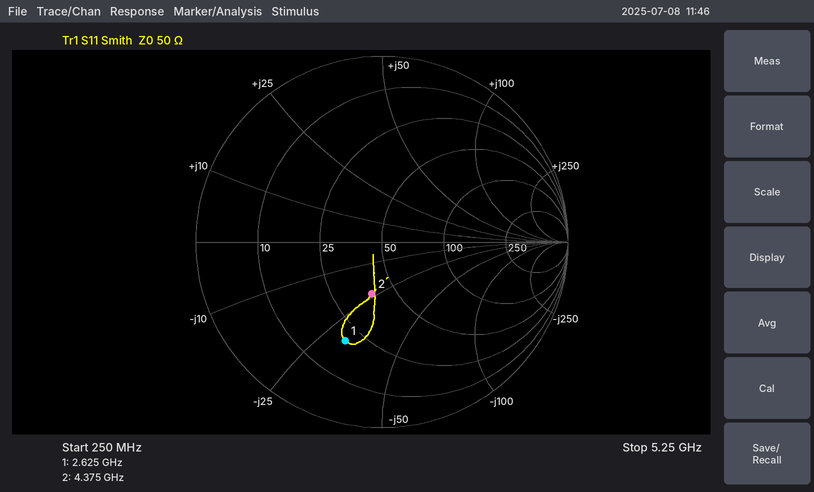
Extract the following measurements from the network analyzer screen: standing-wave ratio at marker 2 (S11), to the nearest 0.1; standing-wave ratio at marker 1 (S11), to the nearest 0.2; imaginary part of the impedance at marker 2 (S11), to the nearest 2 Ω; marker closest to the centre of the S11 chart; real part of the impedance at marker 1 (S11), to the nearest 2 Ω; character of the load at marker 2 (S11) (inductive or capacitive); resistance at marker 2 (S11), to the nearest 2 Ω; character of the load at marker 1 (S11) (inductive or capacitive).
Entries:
1.8
3.6
-24 Ω
marker 2
20 Ω
capacitive
38 Ω
capacitive
